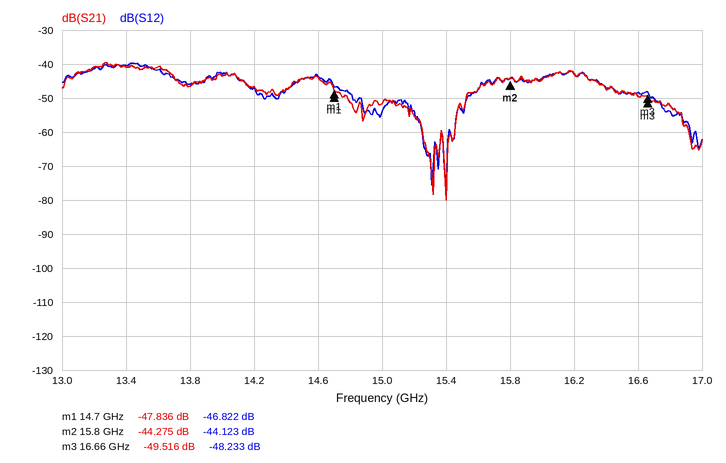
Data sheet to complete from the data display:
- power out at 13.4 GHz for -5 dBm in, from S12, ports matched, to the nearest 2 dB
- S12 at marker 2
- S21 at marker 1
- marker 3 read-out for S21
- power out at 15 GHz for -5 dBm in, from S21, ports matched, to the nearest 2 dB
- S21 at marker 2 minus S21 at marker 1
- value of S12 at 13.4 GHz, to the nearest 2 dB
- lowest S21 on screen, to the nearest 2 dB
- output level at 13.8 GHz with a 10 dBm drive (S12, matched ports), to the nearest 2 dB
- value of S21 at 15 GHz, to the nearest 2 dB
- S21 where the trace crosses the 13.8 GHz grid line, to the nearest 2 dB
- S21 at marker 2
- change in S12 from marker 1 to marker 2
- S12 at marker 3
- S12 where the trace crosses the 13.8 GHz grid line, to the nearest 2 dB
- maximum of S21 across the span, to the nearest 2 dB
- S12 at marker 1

-46 dBm
-44.123 dB
-47.836 dB
-49.516 dB
-56 dBm
3.561 dB
-40 dB
-80 dB
-36 dBm
-52 dB
-46 dB
-44.275 dB
2.699 dB
-48.233 dB
-46 dB
-40 dB
-46.822 dB
